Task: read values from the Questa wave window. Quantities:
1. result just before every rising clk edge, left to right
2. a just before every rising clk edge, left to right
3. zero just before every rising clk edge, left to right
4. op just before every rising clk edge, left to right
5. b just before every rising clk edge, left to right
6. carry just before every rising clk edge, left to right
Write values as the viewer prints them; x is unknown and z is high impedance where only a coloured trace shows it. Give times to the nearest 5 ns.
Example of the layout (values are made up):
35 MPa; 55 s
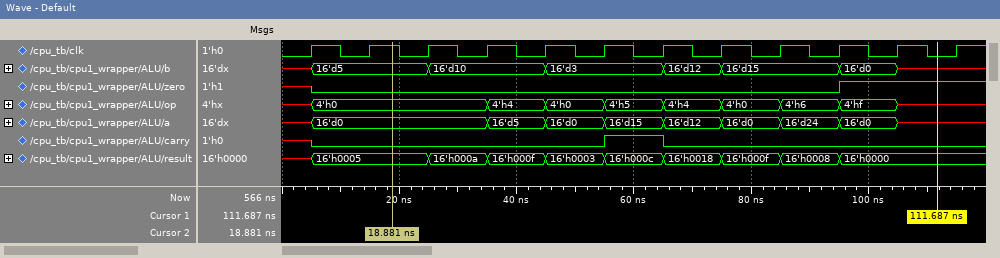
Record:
x, 16'h0005, 16'h0005, 16'h000a, 16'h000f, 16'h0003, 16'h000c, 16'h0018, 16'h000f, 16'h0008, 16'h0000, 16'h0000; x, 16'd0, 16'd0, 16'd0, 16'd5, 16'd0, 16'd15, 16'd12, 16'd0, 16'd24, 16'd0, x; x 0 0 0 0 0 0 0 0 0 1 1; x, 4'h0, 4'h0, 4'h0, 4'h4, 4'h0, 4'h5, 4'h4, 4'h0, 4'h6, 4'hf, x; x, 16'd5, 16'd5, 16'd10, 16'd10, 16'd3, 16'd3, 16'd12, 16'd15, 16'd15, 16'd0, x; x 0 0 0 0 0 1 0 0 0 0 0
